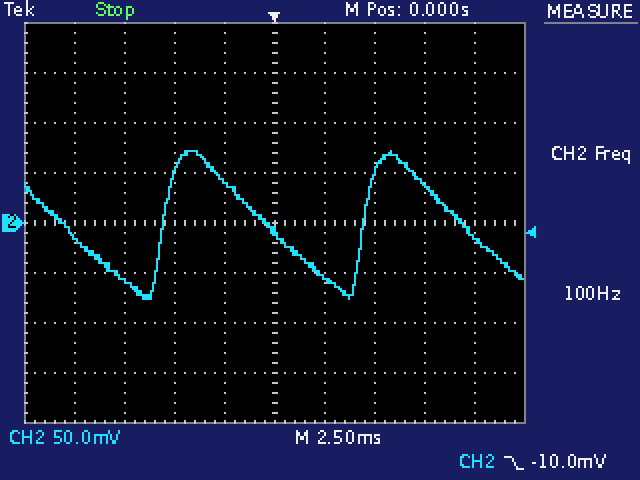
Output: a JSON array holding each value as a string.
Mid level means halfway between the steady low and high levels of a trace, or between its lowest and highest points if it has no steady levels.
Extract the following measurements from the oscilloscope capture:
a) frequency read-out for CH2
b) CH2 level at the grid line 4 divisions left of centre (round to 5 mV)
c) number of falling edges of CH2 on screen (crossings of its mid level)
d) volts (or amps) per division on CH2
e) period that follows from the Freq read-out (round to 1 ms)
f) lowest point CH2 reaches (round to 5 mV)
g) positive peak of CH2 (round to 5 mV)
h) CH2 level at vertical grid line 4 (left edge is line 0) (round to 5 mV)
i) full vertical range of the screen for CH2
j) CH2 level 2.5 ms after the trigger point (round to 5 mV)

["100 Hz", "-15 mV", "3", "50 mV", "10 ms", "-75 mV", "70 mV", "40 mV", "400 mV", "-55 mV"]
